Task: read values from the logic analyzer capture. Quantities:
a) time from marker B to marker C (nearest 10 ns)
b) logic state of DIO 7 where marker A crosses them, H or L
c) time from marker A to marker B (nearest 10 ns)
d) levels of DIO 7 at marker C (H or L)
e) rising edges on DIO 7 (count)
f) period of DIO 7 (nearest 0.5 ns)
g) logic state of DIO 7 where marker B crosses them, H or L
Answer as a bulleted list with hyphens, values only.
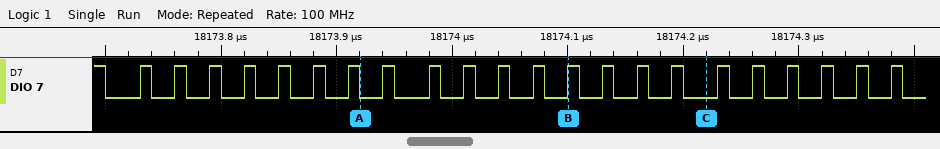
- 120 ns
- DIO 7=L
- 180 ns
- DIO 7=L
- 22
- 31 ns
- DIO 7=H
